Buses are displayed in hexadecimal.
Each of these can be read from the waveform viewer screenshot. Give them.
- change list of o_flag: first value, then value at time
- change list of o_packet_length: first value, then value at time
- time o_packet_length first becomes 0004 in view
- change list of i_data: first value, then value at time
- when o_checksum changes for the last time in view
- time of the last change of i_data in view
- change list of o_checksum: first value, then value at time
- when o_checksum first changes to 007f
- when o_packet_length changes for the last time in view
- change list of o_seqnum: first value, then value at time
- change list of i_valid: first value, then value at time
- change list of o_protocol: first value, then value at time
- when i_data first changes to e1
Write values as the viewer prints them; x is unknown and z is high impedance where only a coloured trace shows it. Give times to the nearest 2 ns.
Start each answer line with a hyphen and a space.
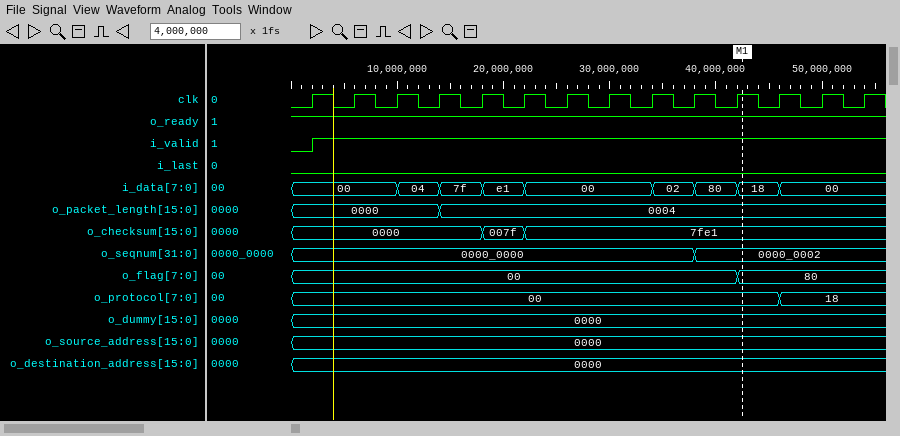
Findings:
- 00, 80 at 42 ns
- 0000, 0004 at 14 ns
- 14 ns
- 00, 04 at 10 ns, 7f at 14 ns, e1 at 18 ns, 00 at 22 ns, 02 at 34 ns, 80 at 38 ns, 18 at 42 ns, 00 at 46 ns
- 22 ns
- 46 ns
- 0000, 007f at 18 ns, 7fe1 at 22 ns
- 18 ns
- 14 ns
- 0000_0000, 0000_0002 at 38 ns
- 0, 1 at 2 ns
- 00, 18 at 46 ns
- 18 ns
